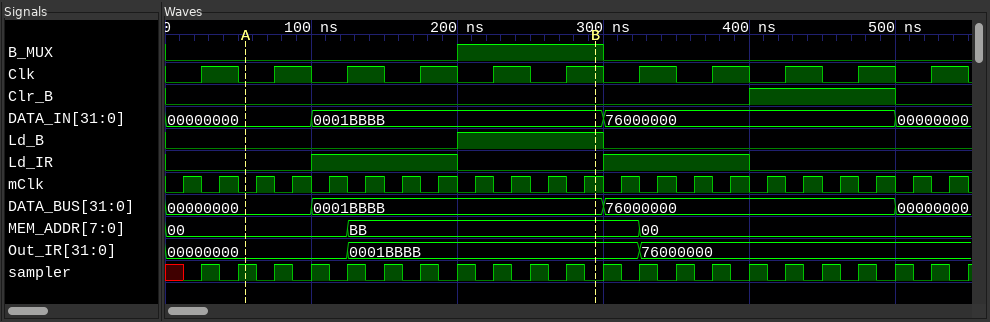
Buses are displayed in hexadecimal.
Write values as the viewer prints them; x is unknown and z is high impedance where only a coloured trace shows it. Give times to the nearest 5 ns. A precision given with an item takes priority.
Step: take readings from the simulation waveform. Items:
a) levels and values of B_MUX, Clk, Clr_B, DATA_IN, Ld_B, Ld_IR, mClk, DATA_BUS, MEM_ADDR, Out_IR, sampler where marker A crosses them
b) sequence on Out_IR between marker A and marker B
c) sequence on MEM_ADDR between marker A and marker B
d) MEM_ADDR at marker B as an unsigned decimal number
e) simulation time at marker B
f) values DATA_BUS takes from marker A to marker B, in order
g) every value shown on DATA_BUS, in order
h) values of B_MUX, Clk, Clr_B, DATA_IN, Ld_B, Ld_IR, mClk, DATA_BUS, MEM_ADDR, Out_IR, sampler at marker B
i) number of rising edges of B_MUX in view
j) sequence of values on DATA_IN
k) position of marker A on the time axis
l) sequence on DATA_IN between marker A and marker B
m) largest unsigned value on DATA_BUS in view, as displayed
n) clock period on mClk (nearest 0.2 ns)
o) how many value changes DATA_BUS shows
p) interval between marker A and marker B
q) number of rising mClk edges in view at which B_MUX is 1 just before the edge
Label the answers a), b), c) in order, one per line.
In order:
a) B_MUX=0, Clk=0, Clr_B=0, DATA_IN=00000000, Ld_B=0, Ld_IR=0, mClk=0, DATA_BUS=00000000, MEM_ADDR=00, Out_IR=00000000, sampler=1
b) 00000000, 0001BBBB
c) 00, BB
d) 187
e) 295 ns
f) 00000000, 0001BBBB
g) 00000000, 0001BBBB, 76000000, 00000000
h) B_MUX=1, Clk=1, Clr_B=0, DATA_IN=0001BBBB, Ld_B=1, Ld_IR=0, mClk=1, DATA_BUS=0001BBBB, MEM_ADDR=BB, Out_IR=0001BBBB, sampler=0
i) 1
j) 00000000, 0001BBBB, 76000000, 00000000
k) 55 ns
l) 00000000, 0001BBBB
m) 76000000
n) 25 ns
o) 3
p) 240 ns
q) 4
